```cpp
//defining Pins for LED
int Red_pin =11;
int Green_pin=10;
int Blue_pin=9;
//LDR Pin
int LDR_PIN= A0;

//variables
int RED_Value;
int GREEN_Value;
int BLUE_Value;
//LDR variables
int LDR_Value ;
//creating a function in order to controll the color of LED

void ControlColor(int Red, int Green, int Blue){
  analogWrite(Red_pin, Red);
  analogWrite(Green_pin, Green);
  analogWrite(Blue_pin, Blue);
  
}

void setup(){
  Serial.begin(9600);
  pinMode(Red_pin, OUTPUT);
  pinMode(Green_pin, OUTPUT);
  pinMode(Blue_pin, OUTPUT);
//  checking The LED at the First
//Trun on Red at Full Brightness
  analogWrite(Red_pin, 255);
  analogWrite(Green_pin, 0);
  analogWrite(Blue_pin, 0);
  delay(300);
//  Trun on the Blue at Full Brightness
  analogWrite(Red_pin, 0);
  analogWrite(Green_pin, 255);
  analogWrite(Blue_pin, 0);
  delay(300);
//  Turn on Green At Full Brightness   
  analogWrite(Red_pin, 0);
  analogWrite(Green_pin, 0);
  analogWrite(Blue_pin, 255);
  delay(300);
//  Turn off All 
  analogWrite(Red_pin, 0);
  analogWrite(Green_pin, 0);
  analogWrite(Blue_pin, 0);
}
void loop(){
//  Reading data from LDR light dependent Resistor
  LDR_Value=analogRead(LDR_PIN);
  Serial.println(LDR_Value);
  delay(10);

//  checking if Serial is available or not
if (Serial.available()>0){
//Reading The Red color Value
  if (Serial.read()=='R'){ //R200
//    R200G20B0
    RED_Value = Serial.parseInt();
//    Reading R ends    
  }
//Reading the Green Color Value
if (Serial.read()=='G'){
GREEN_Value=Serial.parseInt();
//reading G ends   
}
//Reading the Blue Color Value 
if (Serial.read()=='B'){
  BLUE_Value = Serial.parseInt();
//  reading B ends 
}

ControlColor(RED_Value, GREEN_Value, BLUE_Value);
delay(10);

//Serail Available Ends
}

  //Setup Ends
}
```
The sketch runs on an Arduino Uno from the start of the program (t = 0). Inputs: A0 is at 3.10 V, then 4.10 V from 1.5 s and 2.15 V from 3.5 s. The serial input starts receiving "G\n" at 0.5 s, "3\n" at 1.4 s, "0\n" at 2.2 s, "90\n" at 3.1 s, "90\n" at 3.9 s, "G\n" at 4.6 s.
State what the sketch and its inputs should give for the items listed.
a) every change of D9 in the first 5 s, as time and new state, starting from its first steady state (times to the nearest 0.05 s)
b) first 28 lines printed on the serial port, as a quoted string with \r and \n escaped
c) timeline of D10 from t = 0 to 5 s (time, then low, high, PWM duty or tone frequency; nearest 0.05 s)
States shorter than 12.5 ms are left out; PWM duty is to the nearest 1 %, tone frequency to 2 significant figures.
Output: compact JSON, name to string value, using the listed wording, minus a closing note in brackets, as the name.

{"every change of D9 in the first 5 s, as time and new state, starting from its first steady state": "0 s low; 0.6 s high; 0.9 s low", "first 28 lines printed on the serial port, as a quoted string with \\r and \\n escaped": "\"634\\r\\n634\\r\\n634\\r\\n634\\r\\n634\\r\\n634\\r\\n634\\r\\n634\\r\\n634\\r\\n634\\r\\n634\\r\\n634\\r\\n634\\r\\n634\\r\\n634\\r\\n634\\r\\n634\\r\\n634\\r\\n634\\r\\n634\\r\\n634\\r\\n634\\r\\n634\\r\\n634\\r\\n634\\r\\n634\\r\\n634\\r\\n634\\r\\n\"", "timeline of D10 from t = 0 to 5 s": "0 s low; 0.3 s high; 0.6 s low"}
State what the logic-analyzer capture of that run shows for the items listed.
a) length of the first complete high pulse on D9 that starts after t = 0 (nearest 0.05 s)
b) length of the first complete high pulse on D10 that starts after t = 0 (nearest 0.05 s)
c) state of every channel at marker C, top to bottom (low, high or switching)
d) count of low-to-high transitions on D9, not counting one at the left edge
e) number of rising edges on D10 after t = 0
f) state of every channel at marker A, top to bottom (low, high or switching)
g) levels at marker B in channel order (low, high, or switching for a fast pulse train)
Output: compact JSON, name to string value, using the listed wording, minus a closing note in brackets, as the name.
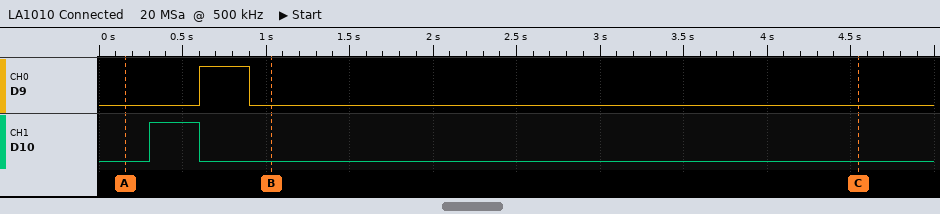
{"length of the first complete high pulse on D9 that starts after t = 0": "0.30 s", "length of the first complete high pulse on D10 that starts after t = 0": "0.30 s", "state of every channel at marker C, top to bottom": "D9 low, D10 low", "count of low-to-high transitions on D9, not counting one at the left edge": "1", "number of rising edges on D10 after t = 0": "1", "state of every channel at marker A, top to bottom": "D9 low, D10 low", "levels at marker B in channel order": "D9 low, D10 low"}
